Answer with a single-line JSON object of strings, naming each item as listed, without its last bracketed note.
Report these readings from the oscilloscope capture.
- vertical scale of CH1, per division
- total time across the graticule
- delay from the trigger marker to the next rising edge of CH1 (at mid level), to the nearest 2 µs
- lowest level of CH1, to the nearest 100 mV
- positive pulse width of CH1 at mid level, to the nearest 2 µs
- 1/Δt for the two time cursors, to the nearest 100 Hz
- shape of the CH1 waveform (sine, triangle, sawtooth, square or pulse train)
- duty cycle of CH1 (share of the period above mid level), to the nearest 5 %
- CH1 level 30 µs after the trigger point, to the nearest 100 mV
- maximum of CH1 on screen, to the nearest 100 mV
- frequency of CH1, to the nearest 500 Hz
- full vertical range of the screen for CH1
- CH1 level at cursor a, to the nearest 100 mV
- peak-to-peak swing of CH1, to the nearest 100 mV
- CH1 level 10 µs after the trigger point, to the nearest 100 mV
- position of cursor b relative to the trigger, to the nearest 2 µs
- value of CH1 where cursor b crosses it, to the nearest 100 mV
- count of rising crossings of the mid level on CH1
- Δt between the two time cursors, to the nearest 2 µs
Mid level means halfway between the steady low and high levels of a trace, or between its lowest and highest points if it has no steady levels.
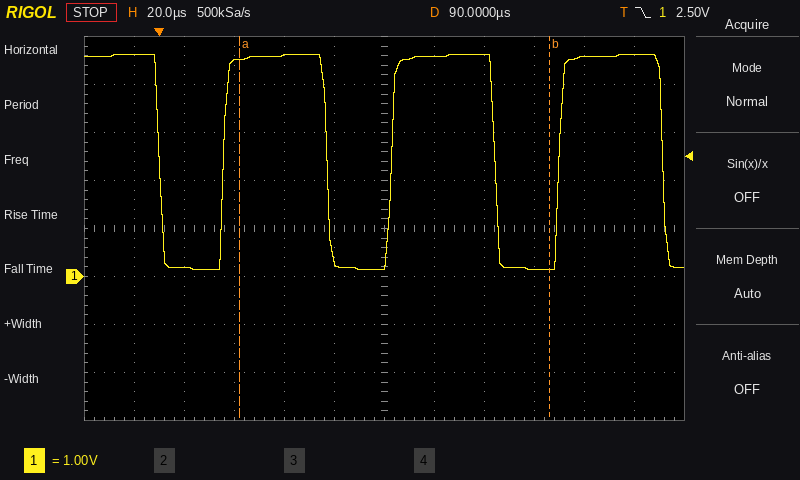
{"vertical scale of CH1, per division": "1 V", "total time across the graticule": "240 µs", "delay from the trigger marker to the next rising edge of CH1 (at mid level), to the nearest 2 µs": "26 µs", "lowest level of CH1, to the nearest 100 mV": "100 mV", "positive pulse width of CH1 at mid level, to the nearest 2 µs": "42 µs", "1/Δt for the two time cursors, to the nearest 100 Hz": "8.1 kHz", "shape of the CH1 waveform": "pulse train", "duty cycle of CH1 (share of the period above mid level), to the nearest 5 %": "60 %", "CH1 level 30 µs after the trigger point, to the nearest 100 mV": "4.5 V", "maximum of CH1 on screen, to the nearest 100 mV": "4.6 V", "frequency of CH1, to the nearest 500 Hz": "15.0 kHz", "full vertical range of the screen for CH1": "8 V", "CH1 level at cursor a, to the nearest 100 mV": "4.5 V", "peak-to-peak swing of CH1, to the nearest 100 mV": "4.5 V", "CH1 level 10 µs after the trigger point, to the nearest 100 mV": "200 mV", "position of cursor b relative to the trigger, to the nearest 2 µs": "+156 µs", "value of CH1 where cursor b crosses it, to the nearest 100 mV": "100 mV", "count of rising crossings of the mid level on CH1": "3", "Δt between the two time cursors, to the nearest 2 µs": "124 µs"}
